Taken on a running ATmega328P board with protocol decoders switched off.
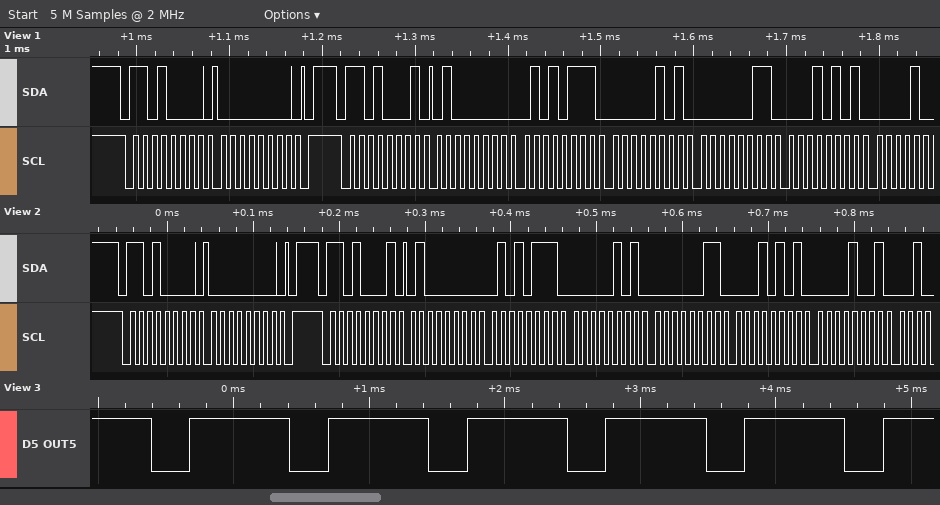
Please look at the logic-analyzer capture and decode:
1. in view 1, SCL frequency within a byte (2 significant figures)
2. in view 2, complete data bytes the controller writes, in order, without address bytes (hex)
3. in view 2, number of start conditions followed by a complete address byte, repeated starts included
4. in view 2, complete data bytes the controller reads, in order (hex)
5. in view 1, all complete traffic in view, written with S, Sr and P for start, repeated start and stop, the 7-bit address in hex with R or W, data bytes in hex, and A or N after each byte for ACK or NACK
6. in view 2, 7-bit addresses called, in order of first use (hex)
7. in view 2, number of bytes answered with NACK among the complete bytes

100 kHz
00
2
40 57 05 03 15 09
S 68W A 00 A P S 68R A 40 A 57 A 05 A 03 A 15 A
0x68
0
